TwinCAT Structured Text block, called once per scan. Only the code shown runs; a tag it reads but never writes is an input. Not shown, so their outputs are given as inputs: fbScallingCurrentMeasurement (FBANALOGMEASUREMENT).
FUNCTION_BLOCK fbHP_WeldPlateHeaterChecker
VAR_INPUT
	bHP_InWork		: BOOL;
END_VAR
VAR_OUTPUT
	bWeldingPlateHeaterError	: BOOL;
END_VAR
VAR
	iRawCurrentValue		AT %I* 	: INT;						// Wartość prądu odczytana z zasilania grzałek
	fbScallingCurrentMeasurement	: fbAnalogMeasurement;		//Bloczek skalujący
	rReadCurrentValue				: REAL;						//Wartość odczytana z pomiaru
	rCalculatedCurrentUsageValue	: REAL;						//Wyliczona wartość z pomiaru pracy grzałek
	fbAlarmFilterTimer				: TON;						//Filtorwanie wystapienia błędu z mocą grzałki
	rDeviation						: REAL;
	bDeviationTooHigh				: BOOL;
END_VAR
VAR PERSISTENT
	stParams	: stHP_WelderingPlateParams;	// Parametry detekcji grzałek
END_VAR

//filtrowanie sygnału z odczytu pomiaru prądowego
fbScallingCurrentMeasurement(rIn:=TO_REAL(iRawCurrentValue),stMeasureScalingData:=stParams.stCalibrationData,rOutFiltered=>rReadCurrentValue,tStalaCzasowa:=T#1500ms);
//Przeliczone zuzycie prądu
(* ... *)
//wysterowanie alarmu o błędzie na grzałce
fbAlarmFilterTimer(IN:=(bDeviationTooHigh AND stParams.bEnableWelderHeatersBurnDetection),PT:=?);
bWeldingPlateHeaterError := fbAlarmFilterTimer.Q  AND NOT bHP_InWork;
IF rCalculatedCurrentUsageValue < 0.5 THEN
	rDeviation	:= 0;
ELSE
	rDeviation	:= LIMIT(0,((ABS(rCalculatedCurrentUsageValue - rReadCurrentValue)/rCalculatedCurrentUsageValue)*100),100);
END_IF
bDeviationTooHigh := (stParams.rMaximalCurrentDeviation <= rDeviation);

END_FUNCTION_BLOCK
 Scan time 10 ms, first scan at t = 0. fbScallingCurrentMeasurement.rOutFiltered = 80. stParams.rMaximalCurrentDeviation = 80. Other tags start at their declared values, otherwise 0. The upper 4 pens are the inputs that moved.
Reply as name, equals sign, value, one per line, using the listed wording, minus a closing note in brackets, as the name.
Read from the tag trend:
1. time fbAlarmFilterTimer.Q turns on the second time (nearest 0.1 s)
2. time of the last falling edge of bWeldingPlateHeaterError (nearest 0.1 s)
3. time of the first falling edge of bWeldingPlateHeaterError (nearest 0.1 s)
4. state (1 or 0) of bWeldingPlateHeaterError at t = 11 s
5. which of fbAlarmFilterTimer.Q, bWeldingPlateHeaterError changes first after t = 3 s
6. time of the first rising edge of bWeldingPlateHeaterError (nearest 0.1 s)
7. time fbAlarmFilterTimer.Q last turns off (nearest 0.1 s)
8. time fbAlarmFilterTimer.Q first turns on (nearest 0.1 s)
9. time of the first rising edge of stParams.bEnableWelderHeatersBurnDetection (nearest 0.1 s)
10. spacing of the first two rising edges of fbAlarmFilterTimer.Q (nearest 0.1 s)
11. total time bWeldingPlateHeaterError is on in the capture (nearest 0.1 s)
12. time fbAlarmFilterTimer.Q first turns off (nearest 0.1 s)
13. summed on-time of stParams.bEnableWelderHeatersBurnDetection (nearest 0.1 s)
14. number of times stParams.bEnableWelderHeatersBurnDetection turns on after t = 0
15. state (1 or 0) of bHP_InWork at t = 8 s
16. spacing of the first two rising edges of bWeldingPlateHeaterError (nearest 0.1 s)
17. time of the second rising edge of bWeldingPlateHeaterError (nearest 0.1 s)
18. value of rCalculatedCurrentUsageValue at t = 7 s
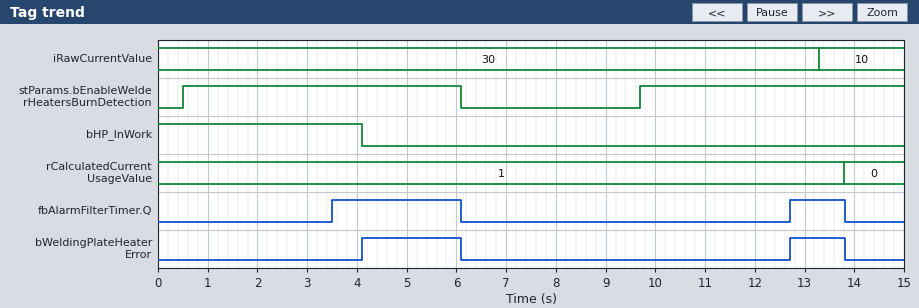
time fbAlarmFilterTimer.Q turns on the second time = 12.7 s
time of the last falling edge of bWeldingPlateHeaterError = 13.8 s
time of the first falling edge of bWeldingPlateHeaterError = 6.1 s
state (1 or 0) of bWeldingPlateHeaterError at t = 11 s = 0
which of fbAlarmFilterTimer.Q, bWeldingPlateHeaterError changes first after t = 3 s = fbAlarmFilterTimer.Q
time of the first rising edge of bWeldingPlateHeaterError = 4.1 s
time fbAlarmFilterTimer.Q last turns off = 13.8 s
time fbAlarmFilterTimer.Q first turns on = 3.5 s
time of the first rising edge of stParams.bEnableWelderHeatersBurnDetection = 0.5 s
spacing of the first two rising edges of fbAlarmFilterTimer.Q = 9.2 s
total time bWeldingPlateHeaterError is on in the capture = 3.1 s
time fbAlarmFilterTimer.Q first turns off = 6.1 s
summed on-time of stParams.bEnableWelderHeatersBurnDetection = 10.9 s
number of times stParams.bEnableWelderHeatersBurnDetection turns on after t = 0 = 2
state (1 or 0) of bHP_InWork at t = 8 s = 0
spacing of the first two rising edges of bWeldingPlateHeaterError = 8.6 s
time of the second rising edge of bWeldingPlateHeaterError = 12.7 s
value of rCalculatedCurrentUsageValue at t = 7 s = 1
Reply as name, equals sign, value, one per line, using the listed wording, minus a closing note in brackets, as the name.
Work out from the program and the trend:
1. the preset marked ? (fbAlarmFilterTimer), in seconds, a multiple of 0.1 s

the preset marked ? (fbAlarmFilterTimer), in seconds, a multiple of 0.1 s = 3.0 s
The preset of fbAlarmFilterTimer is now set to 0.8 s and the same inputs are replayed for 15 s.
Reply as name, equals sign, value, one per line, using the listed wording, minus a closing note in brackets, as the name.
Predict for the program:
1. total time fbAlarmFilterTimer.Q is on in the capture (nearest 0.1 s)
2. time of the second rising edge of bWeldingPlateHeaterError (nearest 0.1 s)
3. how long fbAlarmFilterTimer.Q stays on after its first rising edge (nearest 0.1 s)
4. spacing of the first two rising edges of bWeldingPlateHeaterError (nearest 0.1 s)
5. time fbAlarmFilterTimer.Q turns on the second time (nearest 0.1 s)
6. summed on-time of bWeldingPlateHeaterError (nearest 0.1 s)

total time fbAlarmFilterTimer.Q is on in the capture = 8.1 s
time of the second rising edge of bWeldingPlateHeaterError = 10.5 s
how long fbAlarmFilterTimer.Q stays on after its first rising edge = 4.8 s
spacing of the first two rising edges of bWeldingPlateHeaterError = 6.4 s
time fbAlarmFilterTimer.Q turns on the second time = 10.5 s
summed on-time of bWeldingPlateHeaterError = 5.3 s
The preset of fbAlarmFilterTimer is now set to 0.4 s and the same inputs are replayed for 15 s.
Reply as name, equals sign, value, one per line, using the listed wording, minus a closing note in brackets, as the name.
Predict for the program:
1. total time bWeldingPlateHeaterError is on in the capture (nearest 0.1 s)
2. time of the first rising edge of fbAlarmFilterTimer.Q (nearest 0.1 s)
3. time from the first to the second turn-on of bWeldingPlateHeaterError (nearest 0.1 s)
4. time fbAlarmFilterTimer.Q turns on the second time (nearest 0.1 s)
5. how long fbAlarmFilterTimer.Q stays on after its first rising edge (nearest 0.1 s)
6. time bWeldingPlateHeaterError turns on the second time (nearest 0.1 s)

total time bWeldingPlateHeaterError is on in the capture = 5.7 s
time of the first rising edge of fbAlarmFilterTimer.Q = 0.9 s
time from the first to the second turn-on of bWeldingPlateHeaterError = 6.0 s
time fbAlarmFilterTimer.Q turns on the second time = 10.1 s
how long fbAlarmFilterTimer.Q stays on after its first rising edge = 5.2 s
time bWeldingPlateHeaterError turns on the second time = 10.1 s
